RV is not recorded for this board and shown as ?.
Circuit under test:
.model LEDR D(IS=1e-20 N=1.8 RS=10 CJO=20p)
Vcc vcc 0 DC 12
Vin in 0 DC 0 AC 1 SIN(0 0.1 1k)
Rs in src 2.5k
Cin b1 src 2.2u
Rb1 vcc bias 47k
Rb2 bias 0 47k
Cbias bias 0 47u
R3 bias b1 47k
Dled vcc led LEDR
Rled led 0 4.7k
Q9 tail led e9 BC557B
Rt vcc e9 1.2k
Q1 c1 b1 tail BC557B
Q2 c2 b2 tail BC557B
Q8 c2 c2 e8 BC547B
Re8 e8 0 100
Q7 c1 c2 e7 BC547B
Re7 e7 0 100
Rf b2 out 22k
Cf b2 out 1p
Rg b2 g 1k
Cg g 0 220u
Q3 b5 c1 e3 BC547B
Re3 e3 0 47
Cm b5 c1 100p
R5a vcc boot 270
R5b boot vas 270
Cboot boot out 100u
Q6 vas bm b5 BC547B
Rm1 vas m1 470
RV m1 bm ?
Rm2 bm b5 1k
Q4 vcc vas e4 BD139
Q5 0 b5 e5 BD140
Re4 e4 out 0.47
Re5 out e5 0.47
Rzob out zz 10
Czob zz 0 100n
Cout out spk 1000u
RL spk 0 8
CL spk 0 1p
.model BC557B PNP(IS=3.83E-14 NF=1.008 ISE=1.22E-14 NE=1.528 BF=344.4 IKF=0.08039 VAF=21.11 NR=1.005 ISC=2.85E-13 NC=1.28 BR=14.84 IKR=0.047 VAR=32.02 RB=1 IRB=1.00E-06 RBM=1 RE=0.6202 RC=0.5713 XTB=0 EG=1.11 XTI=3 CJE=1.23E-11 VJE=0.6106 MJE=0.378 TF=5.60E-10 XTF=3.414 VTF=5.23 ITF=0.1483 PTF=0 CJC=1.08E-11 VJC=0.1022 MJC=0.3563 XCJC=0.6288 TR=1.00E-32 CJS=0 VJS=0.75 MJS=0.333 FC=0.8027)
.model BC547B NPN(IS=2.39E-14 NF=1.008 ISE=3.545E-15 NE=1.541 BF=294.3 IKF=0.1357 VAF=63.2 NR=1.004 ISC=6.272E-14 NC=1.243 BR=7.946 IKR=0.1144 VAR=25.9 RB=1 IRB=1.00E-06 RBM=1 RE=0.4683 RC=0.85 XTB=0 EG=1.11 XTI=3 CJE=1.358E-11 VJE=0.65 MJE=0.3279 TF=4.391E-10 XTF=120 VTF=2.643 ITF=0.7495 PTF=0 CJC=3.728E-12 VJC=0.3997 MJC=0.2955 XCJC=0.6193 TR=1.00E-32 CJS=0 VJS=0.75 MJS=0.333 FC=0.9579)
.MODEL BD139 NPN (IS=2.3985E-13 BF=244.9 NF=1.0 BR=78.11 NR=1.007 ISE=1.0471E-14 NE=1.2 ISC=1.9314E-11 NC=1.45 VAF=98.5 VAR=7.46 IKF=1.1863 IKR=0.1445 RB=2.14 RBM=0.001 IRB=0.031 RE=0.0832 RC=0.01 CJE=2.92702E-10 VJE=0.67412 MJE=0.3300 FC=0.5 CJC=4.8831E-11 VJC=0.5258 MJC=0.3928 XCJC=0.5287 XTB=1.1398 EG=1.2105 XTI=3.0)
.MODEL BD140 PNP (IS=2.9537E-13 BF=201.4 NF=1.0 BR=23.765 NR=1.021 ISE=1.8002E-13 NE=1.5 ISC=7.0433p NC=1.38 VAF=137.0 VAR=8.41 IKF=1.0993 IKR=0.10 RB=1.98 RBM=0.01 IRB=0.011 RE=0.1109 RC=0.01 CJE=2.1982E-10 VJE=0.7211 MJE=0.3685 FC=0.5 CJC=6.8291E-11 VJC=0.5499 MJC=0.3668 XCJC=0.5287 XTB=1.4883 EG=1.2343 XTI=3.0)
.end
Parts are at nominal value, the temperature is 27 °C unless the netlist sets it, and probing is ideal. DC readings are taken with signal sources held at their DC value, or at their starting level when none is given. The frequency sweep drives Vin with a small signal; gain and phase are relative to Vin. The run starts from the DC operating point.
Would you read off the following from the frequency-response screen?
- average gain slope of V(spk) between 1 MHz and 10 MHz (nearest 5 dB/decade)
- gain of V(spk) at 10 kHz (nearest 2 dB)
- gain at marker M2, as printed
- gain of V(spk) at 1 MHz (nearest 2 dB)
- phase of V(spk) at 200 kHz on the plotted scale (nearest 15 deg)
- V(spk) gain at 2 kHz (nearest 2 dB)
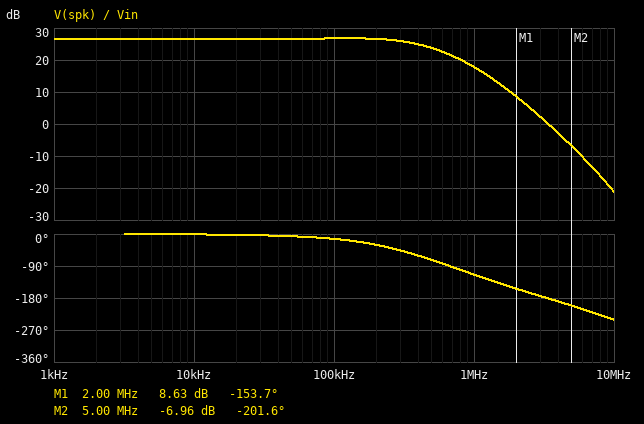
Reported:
-40 dB/decade
26 dB
-6.96 dB
18 dB
-30 deg
26 dB
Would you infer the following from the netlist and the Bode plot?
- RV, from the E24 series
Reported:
180 Ω
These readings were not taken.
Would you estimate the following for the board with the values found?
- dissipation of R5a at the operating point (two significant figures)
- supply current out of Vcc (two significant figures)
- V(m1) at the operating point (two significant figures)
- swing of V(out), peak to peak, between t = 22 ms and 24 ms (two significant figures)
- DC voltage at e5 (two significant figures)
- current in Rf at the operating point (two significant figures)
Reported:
26 mW
15 mA
6.3 V
4.3 V
6.1 V
1.2 µA
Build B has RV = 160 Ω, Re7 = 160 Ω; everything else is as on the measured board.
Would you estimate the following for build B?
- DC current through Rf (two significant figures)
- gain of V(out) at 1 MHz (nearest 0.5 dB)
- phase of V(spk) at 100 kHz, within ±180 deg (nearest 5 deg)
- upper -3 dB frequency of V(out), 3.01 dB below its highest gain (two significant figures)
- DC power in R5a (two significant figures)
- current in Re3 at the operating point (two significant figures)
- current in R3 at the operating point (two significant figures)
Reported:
1.4 µA
14.5 dB
-20 deg
360 kHz
27 mW
10 mA
1.1 µA
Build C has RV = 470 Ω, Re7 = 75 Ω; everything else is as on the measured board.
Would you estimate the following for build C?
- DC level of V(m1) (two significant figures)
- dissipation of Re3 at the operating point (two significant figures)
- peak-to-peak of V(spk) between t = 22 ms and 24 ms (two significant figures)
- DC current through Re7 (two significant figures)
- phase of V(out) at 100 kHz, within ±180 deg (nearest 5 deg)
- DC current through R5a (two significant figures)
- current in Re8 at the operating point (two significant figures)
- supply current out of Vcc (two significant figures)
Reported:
6.4 V
4.4 mW
4.3 V
550 µA
-5 deg
9.7 mA
460 µA
56 mA
